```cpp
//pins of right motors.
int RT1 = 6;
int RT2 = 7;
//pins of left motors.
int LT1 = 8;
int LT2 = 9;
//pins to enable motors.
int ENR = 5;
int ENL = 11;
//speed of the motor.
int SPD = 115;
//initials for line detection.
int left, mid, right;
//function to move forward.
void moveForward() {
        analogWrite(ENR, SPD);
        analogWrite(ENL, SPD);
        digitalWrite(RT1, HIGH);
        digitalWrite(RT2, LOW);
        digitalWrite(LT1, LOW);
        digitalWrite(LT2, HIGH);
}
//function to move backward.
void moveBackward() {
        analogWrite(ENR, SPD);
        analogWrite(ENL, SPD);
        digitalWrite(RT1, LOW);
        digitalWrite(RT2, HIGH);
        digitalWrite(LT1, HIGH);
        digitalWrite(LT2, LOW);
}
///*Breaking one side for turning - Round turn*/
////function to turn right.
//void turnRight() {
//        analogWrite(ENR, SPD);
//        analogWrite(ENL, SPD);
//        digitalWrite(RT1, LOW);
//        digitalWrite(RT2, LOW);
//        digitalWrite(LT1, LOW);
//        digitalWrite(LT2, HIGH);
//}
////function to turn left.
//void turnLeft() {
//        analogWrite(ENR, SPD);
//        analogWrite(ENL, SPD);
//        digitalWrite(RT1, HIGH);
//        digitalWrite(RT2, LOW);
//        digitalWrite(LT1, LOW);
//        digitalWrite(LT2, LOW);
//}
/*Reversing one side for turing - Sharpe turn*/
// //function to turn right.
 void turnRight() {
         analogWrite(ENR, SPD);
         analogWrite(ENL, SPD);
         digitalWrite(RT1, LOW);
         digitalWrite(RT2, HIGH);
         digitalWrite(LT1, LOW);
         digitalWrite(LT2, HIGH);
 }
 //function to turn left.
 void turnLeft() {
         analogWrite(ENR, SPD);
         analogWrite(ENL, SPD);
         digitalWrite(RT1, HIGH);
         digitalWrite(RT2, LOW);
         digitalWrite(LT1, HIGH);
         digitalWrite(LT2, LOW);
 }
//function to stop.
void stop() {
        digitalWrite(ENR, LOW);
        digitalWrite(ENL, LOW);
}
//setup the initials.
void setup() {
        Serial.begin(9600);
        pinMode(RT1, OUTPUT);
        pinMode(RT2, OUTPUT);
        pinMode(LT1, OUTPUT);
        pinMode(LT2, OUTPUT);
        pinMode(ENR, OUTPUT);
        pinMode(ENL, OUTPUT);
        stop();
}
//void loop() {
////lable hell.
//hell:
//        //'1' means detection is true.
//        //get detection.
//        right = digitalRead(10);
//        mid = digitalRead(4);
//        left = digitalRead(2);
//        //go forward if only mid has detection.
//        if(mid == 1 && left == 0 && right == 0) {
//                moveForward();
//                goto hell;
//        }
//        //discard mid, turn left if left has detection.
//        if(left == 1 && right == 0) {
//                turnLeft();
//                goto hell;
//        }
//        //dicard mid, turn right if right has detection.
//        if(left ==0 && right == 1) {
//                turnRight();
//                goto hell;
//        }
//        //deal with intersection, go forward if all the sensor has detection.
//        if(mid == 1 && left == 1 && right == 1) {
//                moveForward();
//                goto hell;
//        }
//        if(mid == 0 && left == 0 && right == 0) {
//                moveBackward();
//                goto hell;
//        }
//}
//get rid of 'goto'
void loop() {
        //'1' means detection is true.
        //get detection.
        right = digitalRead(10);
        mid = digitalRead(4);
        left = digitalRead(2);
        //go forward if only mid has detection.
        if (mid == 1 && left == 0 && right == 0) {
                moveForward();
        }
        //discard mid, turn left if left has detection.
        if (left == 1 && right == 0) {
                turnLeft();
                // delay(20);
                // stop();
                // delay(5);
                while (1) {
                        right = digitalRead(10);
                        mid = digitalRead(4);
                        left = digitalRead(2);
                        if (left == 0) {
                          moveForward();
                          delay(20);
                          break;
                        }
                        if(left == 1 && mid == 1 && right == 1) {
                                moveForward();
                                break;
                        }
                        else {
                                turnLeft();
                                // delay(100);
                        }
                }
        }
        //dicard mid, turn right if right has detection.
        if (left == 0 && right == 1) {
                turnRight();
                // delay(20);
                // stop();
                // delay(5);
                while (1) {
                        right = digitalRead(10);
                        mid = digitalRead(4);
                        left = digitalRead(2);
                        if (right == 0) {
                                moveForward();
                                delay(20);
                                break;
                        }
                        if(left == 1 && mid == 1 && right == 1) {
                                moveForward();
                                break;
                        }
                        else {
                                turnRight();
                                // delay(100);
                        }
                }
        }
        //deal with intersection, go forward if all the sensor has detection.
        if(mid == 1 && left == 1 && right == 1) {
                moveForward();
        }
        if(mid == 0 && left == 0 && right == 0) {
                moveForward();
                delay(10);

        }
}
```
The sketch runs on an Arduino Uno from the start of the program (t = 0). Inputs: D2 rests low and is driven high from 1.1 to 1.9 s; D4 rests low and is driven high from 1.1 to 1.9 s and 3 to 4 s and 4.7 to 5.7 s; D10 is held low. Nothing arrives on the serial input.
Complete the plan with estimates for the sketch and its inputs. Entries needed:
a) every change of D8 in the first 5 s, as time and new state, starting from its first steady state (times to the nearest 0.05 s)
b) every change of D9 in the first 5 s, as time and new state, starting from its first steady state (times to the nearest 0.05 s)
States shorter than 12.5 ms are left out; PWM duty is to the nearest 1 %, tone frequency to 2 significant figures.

0 s low; 1.1 s high; 1.9 s low
0 s high; 1.1 s low; 1.9 s high
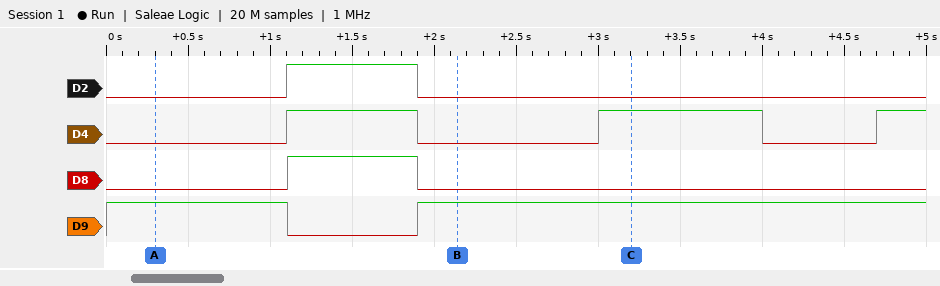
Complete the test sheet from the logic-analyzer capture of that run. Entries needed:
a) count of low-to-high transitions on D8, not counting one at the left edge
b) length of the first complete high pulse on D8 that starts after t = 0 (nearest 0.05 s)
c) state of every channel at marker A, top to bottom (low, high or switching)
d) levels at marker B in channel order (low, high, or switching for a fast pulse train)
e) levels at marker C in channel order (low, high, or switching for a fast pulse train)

1
0.80 s
D2 low, D4 low, D8 low, D9 high
D2 low, D4 low, D8 low, D9 high
D2 low, D4 high, D8 low, D9 high
